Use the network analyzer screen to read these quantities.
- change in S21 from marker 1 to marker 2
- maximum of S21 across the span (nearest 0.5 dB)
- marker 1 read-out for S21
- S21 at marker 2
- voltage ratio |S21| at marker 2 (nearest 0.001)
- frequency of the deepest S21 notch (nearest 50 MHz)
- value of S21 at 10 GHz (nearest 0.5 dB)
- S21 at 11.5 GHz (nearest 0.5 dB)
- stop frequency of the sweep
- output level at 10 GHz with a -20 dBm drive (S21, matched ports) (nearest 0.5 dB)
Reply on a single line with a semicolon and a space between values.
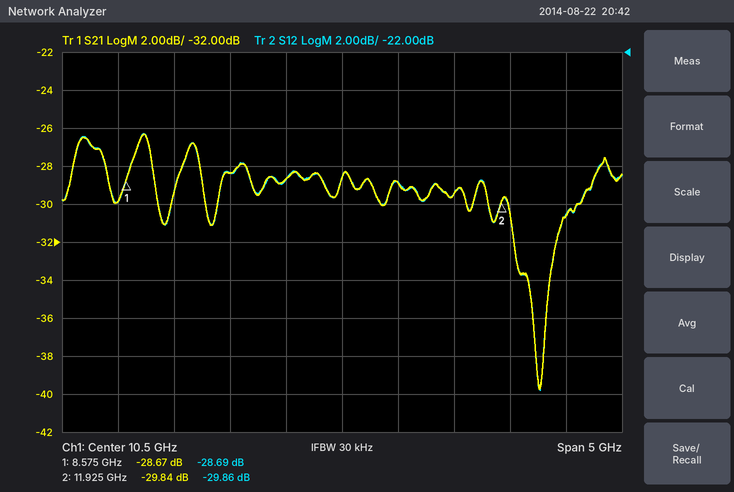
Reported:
-1.17 dB; -26.5 dB; -28.67 dB; -29.84 dB; 0.032; 12.25 GHz; -28.5 dB; -29.5 dB; 13 GHz; -48.5 dBm
